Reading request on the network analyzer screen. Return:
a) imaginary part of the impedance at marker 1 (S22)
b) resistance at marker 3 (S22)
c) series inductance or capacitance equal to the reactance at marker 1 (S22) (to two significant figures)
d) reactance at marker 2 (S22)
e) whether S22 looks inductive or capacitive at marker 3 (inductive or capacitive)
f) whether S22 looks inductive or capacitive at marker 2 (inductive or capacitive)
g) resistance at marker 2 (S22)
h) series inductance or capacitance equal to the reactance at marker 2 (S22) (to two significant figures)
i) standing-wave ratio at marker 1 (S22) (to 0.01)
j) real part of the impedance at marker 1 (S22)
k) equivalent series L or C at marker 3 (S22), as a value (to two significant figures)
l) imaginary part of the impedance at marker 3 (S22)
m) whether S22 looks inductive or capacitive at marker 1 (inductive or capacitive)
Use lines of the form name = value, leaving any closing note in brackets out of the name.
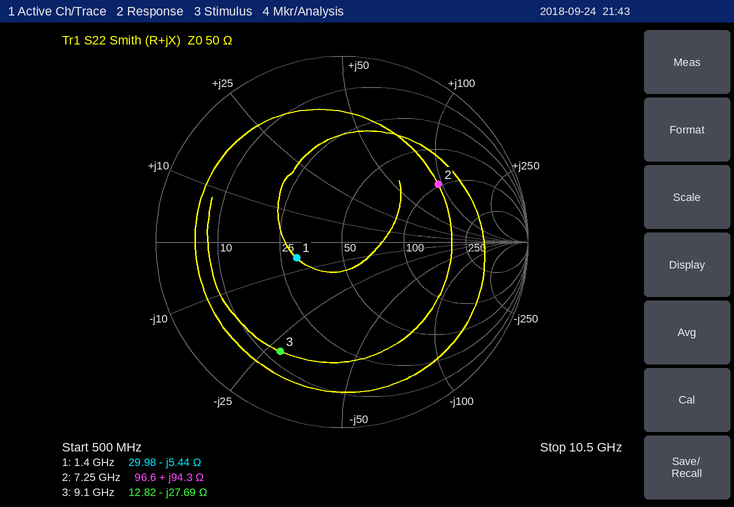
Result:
imaginary part of the impedance at marker 1 = -5.44 Ω
resistance at marker 3 = 12.82 Ω
series inductance or capacitance equal to the reactance at marker 1 (S22) = 21 pF
reactance at marker 2 = +94.3 Ω
whether S22 looks inductive or capacitive at marker 3 = capacitive
whether S22 looks inductive or capacitive at marker 2 = inductive
resistance at marker 2 = 96.6 Ω
series inductance or capacitance equal to the reactance at marker 2 (S22) = 2.1 nH
standing-wave ratio at marker 1 (S22) = 1.70
real part of the impedance at marker 1 = 29.98 Ω
equivalent series L or C at marker 3 (S22), as a value = 630 fF
imaginary part of the impedance at marker 3 = -27.69 Ω
whether S22 looks inductive or capacitive at marker 1 = capacitive
